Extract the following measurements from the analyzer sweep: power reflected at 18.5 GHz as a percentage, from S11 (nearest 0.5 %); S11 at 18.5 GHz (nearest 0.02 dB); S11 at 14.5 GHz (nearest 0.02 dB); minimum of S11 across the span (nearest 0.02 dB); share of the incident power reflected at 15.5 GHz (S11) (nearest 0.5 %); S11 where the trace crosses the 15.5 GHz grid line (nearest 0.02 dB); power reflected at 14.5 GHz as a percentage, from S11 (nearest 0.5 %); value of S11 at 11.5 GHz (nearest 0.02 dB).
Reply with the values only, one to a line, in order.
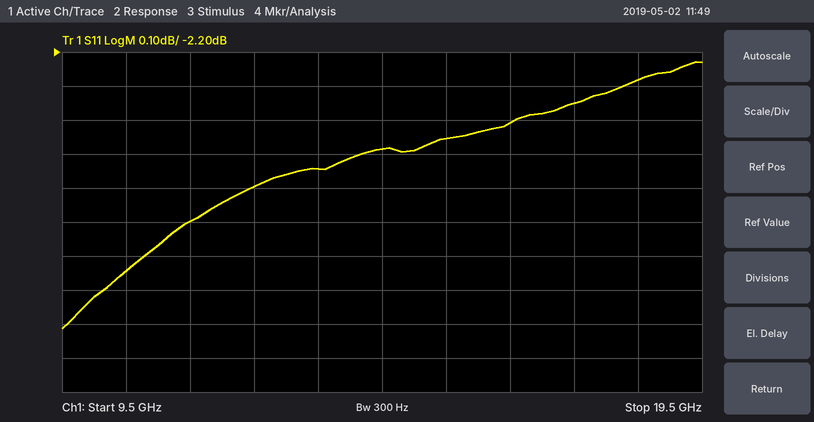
59.0 %
-2.28 dB
-2.48 dB
-3.02 dB
57.0 %
-2.46 dB
56.5 %
-2.70 dB
